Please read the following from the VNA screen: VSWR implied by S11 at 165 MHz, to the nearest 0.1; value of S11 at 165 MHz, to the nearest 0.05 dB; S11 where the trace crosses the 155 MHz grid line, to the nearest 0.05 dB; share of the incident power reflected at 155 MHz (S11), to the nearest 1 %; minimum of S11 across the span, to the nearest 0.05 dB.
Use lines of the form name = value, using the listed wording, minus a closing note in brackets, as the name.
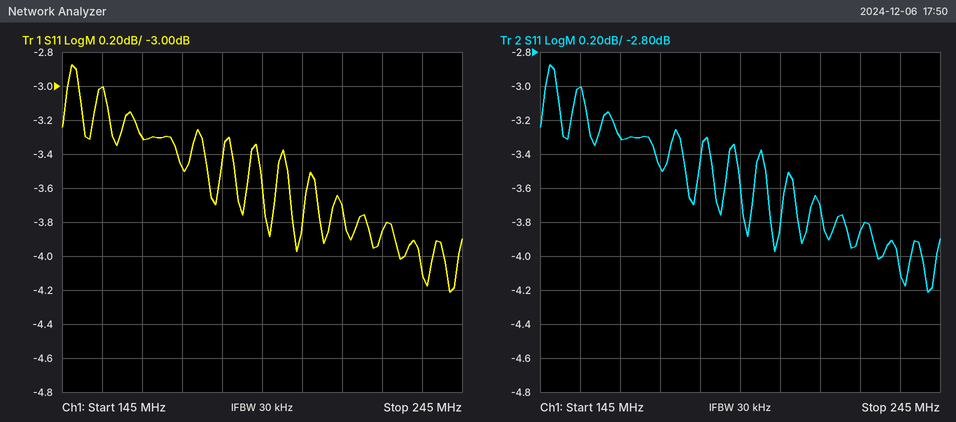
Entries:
VSWR implied by S11 at 165 MHz, to the nearest 0.1 = 5.3
value of S11 at 165 MHz, to the nearest 0.05 dB = -3.30 dB
S11 where the trace crosses the 155 MHz grid line, to the nearest 0.05 dB = -3.00 dB
share of the incident power reflected at 155 MHz (S11), to the nearest 1 % = 50 %
minimum of S11 across the span, to the nearest 0.05 dB = -4.20 dB
